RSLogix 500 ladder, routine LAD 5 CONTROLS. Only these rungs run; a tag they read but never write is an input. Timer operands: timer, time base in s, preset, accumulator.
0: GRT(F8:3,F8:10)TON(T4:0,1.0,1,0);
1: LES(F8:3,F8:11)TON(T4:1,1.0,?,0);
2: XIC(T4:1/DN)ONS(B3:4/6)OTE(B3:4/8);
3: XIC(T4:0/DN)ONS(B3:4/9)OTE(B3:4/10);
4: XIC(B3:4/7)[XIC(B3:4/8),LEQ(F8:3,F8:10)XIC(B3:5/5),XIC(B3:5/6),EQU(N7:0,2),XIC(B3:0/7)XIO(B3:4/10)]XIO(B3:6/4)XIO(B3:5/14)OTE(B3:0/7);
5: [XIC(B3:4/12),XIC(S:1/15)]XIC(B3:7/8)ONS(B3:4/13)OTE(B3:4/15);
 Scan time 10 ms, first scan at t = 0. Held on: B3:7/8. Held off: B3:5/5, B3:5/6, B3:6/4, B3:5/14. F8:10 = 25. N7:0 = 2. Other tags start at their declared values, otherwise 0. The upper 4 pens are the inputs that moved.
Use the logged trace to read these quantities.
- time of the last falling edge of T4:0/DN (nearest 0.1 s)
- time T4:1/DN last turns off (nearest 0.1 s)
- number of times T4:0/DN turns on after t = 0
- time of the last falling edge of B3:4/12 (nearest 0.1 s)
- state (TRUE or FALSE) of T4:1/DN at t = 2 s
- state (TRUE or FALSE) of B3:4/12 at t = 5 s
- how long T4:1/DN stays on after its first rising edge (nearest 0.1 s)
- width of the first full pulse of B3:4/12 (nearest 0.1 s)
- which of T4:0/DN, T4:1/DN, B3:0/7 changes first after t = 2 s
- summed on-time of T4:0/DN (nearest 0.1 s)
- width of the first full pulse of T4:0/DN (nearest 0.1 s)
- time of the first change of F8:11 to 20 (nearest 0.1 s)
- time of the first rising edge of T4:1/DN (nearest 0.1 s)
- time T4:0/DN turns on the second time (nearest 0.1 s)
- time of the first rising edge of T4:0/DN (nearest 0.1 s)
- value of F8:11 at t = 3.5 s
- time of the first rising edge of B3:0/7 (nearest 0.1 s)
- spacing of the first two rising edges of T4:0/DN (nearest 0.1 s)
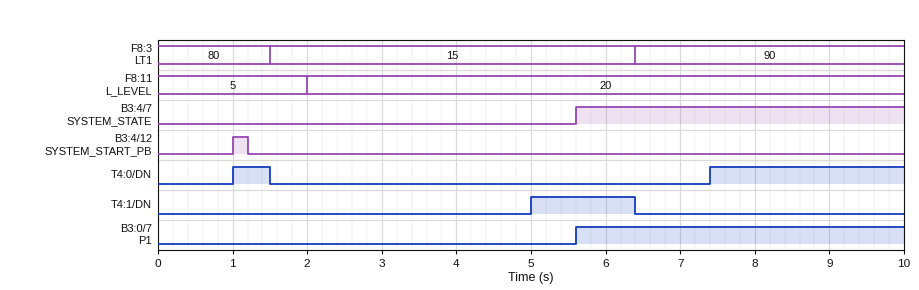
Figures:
1.5 s
6.4 s
2
1.2 s
FALSE
FALSE
1.4 s
0.2 s
T4:1/DN
3.1 s
0.5 s
2.0 s
5.0 s
7.4 s
1.0 s
20
5.6 s
6.4 s
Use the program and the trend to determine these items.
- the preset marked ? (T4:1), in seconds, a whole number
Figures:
3 s
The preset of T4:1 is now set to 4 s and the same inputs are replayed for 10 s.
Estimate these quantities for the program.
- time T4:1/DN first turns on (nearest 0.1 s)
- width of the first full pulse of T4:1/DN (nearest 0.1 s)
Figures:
6.0 s
0.4 s
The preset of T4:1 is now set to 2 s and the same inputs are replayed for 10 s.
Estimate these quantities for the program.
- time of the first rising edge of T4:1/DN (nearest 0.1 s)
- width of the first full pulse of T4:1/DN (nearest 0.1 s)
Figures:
4.0 s
2.4 s
